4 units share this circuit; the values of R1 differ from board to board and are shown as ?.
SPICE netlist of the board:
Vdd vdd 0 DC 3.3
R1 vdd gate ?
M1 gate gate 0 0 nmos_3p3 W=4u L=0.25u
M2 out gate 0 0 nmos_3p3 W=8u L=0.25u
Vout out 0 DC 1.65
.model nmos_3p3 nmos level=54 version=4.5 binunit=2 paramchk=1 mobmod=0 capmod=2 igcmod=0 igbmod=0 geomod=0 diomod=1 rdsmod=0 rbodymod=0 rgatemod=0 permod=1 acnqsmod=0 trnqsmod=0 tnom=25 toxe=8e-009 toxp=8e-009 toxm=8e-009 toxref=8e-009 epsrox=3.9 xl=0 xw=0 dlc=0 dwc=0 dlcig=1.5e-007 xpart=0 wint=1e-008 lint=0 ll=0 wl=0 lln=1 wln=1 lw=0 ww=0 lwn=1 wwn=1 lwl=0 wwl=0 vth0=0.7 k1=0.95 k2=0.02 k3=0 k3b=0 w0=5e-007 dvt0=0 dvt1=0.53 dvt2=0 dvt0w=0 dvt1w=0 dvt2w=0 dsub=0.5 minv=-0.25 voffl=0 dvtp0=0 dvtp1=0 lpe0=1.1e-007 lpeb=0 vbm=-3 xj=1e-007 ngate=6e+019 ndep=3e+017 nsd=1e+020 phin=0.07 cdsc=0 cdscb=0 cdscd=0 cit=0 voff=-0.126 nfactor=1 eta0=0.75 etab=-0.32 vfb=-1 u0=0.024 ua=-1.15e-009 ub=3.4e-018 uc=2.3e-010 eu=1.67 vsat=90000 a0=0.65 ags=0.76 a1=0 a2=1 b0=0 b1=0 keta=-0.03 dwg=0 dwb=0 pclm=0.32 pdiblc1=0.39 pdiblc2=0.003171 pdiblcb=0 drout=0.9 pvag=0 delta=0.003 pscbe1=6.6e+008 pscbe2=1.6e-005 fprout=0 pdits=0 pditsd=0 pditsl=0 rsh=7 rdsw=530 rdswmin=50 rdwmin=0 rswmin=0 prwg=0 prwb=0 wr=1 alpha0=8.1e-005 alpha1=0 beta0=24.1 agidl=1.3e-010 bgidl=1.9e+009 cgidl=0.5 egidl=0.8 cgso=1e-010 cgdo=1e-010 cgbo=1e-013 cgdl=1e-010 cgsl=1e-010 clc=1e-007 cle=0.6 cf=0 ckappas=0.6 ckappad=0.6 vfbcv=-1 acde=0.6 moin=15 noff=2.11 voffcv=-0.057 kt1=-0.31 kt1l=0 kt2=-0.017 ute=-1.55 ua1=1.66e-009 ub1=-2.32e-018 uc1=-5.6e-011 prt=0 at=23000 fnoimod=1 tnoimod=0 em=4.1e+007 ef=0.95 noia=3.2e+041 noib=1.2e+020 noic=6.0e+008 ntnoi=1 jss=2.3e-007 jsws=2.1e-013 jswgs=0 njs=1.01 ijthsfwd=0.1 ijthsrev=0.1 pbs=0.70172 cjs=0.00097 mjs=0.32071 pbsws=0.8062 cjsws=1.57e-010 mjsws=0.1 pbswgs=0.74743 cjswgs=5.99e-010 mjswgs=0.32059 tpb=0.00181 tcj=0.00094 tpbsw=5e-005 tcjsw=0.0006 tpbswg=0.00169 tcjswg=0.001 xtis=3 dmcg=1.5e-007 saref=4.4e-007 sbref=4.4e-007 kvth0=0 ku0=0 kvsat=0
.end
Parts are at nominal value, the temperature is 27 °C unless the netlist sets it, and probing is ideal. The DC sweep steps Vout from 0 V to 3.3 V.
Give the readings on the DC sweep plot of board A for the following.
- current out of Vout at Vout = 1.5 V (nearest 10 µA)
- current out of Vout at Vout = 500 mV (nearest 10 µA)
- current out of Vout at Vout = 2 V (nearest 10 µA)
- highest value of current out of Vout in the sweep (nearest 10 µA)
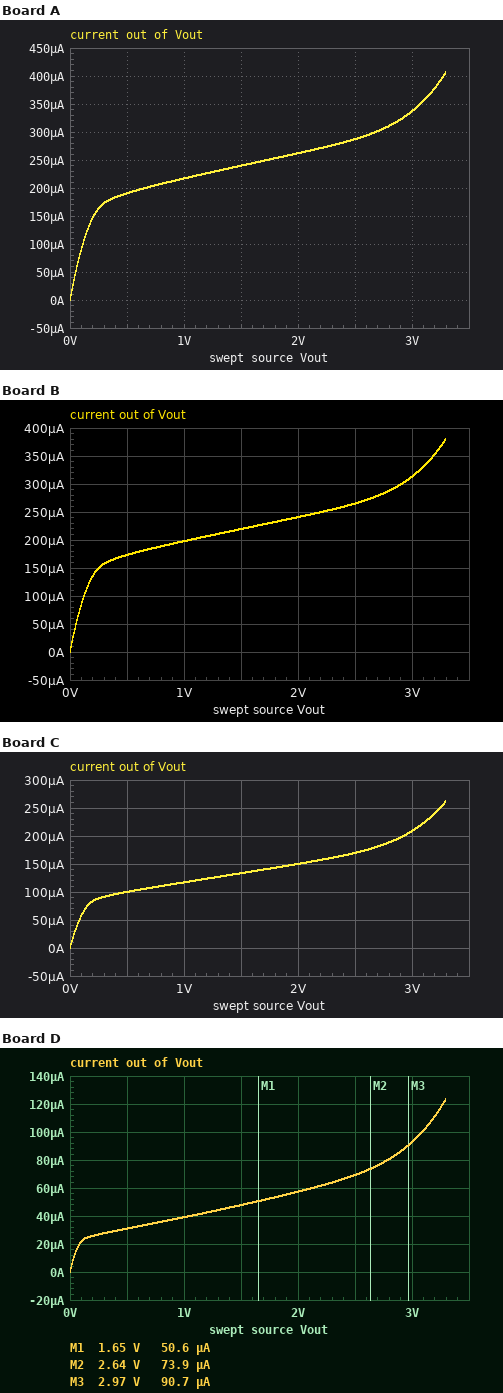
240 µA
190 µA
260 µA
410 µA
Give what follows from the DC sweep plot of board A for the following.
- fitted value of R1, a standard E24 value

18 kΩ
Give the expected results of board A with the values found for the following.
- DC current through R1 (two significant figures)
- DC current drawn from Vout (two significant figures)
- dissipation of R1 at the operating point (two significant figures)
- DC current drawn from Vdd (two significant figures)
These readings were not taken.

110 µA
250 µA
230 µW
110 µA
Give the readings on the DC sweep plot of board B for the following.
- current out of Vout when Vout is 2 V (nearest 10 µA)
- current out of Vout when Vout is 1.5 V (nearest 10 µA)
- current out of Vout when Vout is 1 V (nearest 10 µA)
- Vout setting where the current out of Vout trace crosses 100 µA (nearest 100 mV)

240 µA
220 µA
200 µA
100 mV
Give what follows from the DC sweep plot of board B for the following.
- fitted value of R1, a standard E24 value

20 kΩ
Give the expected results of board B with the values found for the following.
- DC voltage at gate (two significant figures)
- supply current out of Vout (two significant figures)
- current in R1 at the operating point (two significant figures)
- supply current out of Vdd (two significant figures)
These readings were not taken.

1.2 V
230 µA
100 µA
100 µA
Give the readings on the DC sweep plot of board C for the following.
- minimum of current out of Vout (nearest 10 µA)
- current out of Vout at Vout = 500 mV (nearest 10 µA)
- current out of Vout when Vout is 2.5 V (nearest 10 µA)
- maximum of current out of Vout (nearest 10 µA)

0 A
100 µA
170 µA
260 µA
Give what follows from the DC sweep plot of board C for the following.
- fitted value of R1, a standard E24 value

36 kΩ
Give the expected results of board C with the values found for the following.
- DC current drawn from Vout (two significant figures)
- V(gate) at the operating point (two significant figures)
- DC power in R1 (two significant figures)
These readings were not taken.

140 µA
1.1 V
130 µW
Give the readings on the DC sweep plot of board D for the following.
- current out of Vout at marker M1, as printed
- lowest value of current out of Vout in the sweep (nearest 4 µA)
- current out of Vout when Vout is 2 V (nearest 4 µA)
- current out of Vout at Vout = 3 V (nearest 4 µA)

50.6 µA
0 A
56 µA
92 µA
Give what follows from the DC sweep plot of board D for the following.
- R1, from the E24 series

120 kΩ
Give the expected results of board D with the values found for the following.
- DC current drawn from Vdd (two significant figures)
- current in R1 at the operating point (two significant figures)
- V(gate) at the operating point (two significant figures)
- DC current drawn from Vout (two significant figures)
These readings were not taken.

19 µA
19 µA
980 mV
51 µA
